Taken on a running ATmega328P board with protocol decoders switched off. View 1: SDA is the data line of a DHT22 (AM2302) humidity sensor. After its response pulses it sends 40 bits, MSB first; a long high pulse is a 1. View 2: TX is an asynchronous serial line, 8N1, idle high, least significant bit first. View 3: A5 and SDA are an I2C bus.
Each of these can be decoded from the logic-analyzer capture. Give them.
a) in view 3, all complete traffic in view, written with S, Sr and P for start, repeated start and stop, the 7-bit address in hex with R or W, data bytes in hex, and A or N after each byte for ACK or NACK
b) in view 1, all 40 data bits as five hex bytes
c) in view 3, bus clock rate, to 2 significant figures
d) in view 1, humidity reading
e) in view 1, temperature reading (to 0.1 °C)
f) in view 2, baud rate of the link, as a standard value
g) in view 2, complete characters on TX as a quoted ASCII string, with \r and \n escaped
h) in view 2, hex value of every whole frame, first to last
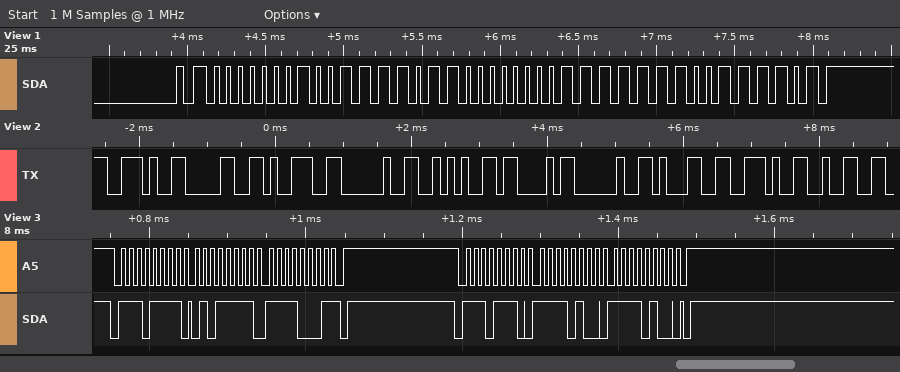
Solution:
S 77R A 5F A F1 N P S 77W A F4 A F4 A P
01 3D 80 7F 3D
100 kHz
31.7 %
-12.7 °C
9600 baud
".09 *C 1.2"
2E 30 39 20 2A 43 20 31 2E 32
